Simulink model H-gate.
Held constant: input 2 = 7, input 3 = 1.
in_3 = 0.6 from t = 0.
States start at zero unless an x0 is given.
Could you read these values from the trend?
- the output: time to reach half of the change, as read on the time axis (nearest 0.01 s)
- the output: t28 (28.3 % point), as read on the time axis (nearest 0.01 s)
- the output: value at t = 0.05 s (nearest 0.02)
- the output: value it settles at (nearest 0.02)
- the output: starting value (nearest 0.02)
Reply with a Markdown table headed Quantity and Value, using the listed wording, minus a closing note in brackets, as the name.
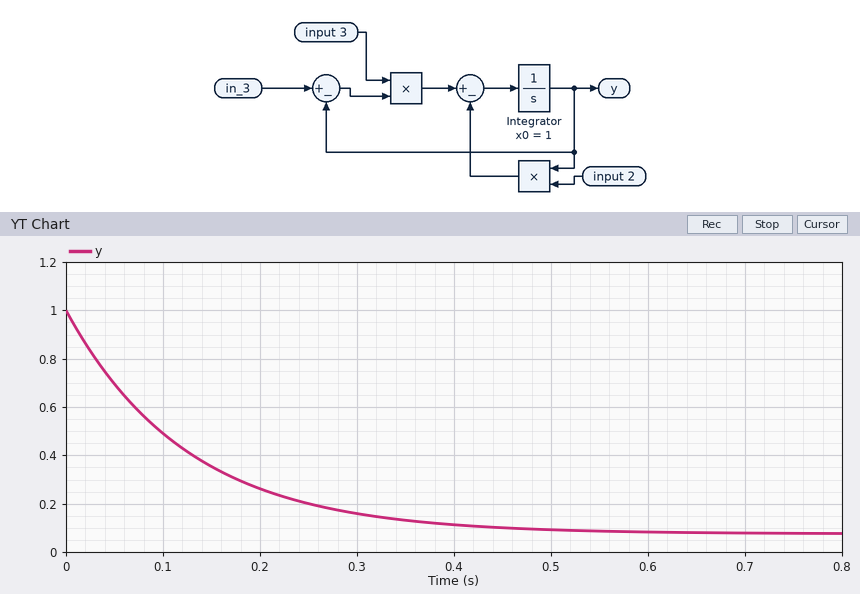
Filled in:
| Quantity | Value |
|---|---|
| the output: time to reach half of the change, as read on the time axis | 0.09 s |
| the output: t28 (28.3 % point), as read on the time axis | 0.04 s |
| the output: value at t = 0.05 s | 0.70 |
| the output: value it settles at | 0.08 |
| the output: starting value | 1.00 |
